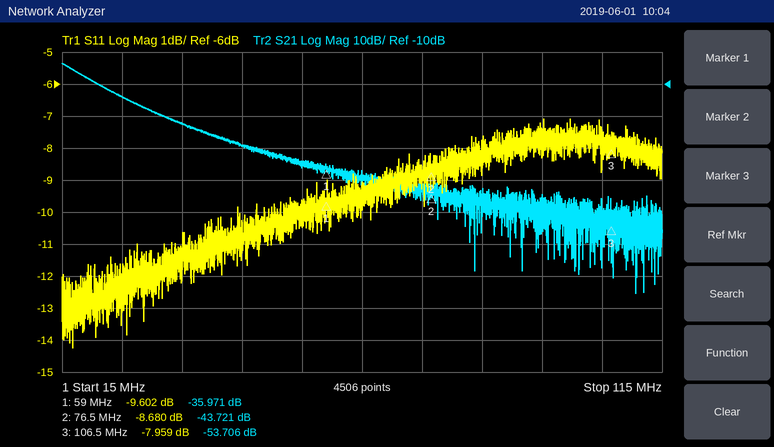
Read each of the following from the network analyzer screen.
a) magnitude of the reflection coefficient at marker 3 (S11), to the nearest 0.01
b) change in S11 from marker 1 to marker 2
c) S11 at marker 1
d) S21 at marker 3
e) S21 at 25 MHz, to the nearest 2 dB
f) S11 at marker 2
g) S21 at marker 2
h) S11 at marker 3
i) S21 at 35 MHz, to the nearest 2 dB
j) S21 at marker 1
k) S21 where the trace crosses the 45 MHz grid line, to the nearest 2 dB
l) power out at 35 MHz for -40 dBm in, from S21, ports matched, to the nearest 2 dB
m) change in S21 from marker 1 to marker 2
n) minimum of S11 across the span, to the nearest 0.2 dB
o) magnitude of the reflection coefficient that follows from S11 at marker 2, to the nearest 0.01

0.40
0.922 dB
-9.602 dB
-53.706 dB
-14 dB
-8.680 dB
-43.721 dB
-7.959 dB
-22 dB
-35.971 dB
-30 dB
-62 dBm
-7.750 dB
-14.2 dB
0.37
